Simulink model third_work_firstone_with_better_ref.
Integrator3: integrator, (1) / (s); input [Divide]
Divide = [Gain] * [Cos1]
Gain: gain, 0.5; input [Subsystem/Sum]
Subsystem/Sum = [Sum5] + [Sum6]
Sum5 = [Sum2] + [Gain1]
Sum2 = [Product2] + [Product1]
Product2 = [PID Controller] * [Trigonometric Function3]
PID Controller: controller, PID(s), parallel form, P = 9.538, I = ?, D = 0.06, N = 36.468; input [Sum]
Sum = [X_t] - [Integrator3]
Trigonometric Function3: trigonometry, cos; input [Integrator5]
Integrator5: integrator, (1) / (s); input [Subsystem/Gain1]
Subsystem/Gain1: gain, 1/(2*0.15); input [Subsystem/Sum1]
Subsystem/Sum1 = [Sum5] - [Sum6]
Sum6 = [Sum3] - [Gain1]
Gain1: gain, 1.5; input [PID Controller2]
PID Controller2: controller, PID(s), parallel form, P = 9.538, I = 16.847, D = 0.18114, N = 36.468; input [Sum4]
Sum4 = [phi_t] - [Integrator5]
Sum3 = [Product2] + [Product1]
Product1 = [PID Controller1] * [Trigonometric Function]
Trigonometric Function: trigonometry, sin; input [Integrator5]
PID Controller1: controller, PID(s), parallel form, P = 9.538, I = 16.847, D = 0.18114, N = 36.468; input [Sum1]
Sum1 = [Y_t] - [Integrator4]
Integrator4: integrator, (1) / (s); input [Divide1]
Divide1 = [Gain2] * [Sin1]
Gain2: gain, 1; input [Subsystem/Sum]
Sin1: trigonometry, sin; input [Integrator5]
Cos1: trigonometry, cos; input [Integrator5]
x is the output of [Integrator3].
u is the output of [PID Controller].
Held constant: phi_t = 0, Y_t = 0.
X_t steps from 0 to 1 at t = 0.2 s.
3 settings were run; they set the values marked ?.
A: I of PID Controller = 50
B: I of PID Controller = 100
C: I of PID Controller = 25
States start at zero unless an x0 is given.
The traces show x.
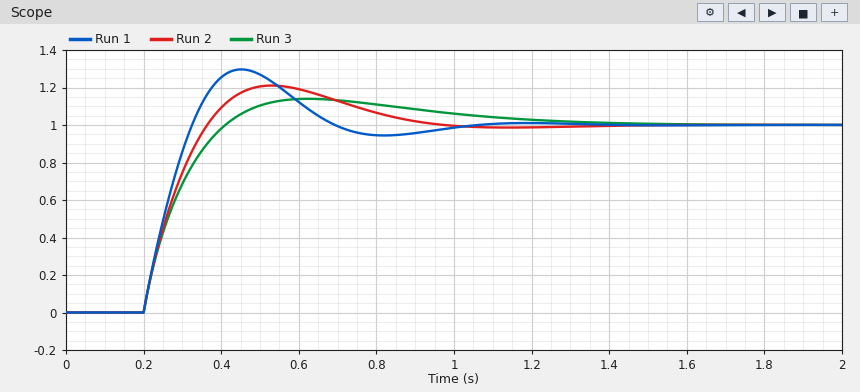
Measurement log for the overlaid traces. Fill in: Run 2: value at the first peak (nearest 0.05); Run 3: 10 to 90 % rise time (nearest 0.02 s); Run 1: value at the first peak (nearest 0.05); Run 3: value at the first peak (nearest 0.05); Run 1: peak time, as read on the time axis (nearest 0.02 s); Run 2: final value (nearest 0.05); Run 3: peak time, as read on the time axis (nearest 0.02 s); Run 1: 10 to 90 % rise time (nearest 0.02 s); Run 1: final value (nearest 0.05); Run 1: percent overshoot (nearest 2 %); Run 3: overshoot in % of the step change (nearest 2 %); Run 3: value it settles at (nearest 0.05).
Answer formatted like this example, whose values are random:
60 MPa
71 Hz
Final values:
1.20
0.16 s
1.30
1.15
0.46 s
1.00
0.62 s
0.10 s
1.00
30 %
14 %
1.00
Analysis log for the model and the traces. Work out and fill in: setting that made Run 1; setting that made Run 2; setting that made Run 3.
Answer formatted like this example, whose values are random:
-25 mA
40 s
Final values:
B
A
C
